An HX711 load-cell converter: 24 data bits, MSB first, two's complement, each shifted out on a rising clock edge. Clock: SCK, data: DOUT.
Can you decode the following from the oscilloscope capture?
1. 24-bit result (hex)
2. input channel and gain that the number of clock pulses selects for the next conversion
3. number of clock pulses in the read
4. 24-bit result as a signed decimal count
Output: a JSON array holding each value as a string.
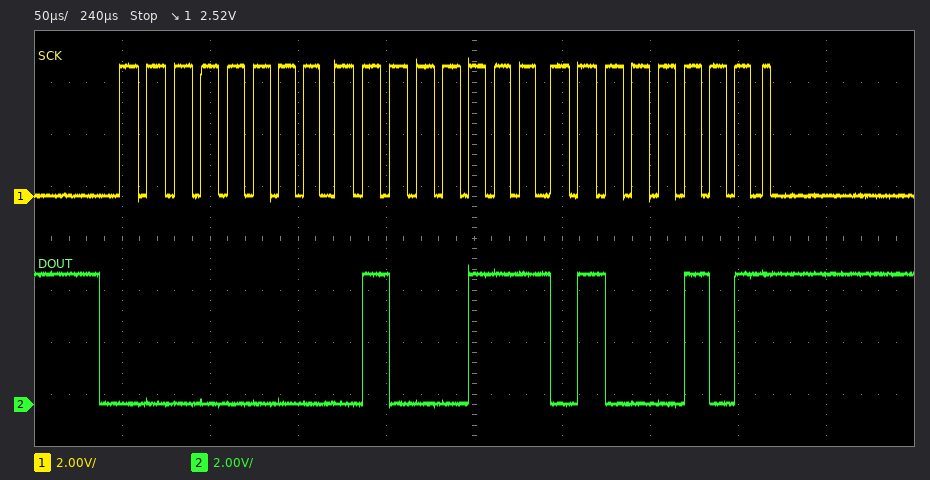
["0x004745", "channel A, gain 128", "25", "18245"]
